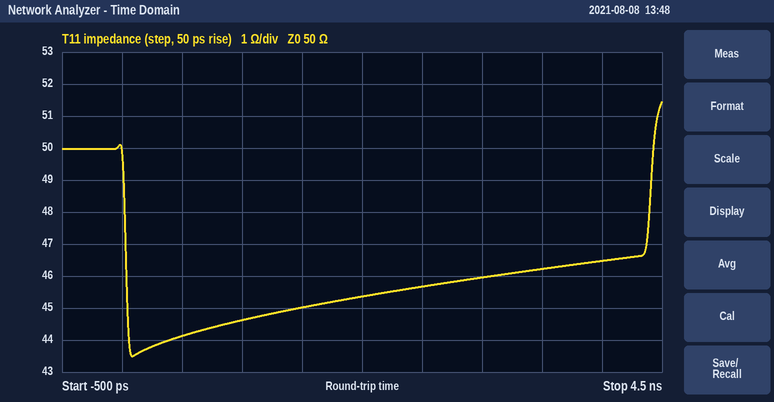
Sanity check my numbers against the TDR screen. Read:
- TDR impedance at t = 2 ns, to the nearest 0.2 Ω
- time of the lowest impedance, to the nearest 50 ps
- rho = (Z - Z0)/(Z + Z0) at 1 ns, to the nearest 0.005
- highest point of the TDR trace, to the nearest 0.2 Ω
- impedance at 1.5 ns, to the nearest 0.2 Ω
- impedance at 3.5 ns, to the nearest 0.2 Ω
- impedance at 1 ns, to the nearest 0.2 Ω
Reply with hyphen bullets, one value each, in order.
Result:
- 45.4 Ω
- 100 ps
- -0.055
- 51.4 Ω
- 45.0 Ω
- 46.2 Ω
- 44.6 Ω
